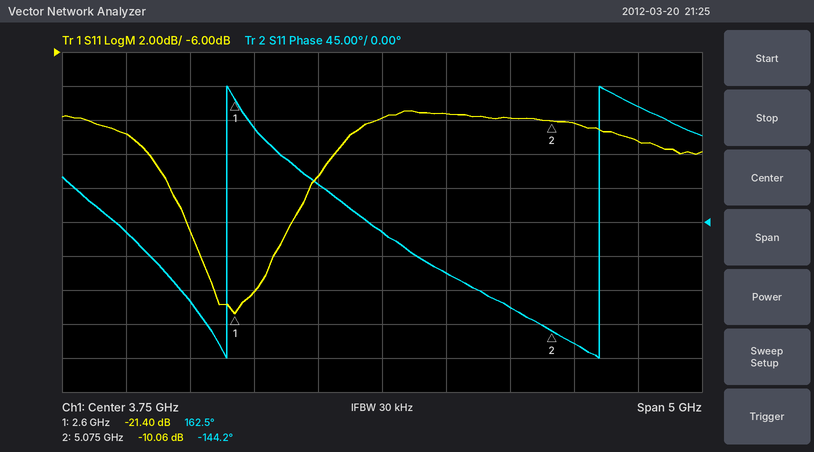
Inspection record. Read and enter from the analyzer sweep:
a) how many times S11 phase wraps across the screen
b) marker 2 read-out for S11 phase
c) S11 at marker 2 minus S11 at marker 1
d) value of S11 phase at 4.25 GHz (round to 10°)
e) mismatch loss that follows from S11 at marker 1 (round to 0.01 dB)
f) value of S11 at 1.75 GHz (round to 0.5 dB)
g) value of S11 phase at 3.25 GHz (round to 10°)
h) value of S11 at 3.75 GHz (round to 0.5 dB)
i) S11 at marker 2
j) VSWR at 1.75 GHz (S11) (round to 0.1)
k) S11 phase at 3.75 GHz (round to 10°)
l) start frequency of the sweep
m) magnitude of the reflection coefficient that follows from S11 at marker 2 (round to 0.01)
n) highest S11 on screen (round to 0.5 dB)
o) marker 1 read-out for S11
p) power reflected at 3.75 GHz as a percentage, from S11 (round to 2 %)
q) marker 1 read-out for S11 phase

2
-144.2°
11.34 dB
-70°
0.03 dB
-11.0 dB
50°
-10.0 dB
-10.06 dB
1.8
-10°
1.25 GHz
0.31
-9.5 dB
-21.40 dB
10 %
162.5°
